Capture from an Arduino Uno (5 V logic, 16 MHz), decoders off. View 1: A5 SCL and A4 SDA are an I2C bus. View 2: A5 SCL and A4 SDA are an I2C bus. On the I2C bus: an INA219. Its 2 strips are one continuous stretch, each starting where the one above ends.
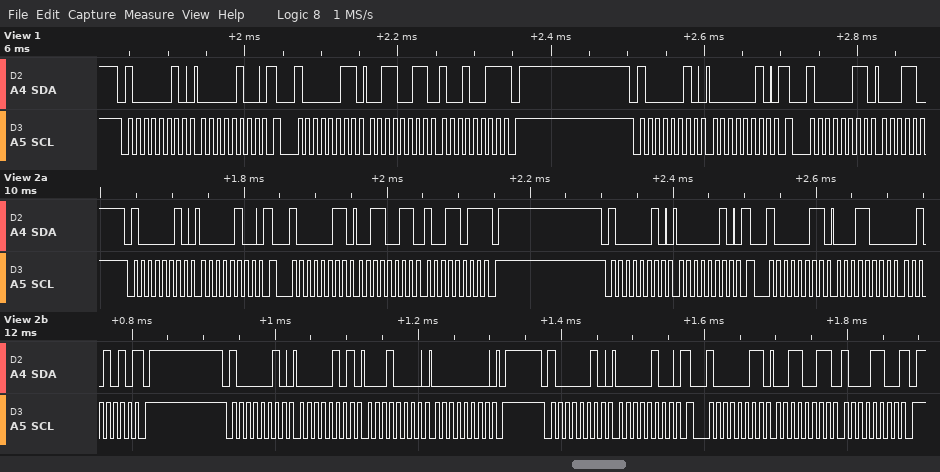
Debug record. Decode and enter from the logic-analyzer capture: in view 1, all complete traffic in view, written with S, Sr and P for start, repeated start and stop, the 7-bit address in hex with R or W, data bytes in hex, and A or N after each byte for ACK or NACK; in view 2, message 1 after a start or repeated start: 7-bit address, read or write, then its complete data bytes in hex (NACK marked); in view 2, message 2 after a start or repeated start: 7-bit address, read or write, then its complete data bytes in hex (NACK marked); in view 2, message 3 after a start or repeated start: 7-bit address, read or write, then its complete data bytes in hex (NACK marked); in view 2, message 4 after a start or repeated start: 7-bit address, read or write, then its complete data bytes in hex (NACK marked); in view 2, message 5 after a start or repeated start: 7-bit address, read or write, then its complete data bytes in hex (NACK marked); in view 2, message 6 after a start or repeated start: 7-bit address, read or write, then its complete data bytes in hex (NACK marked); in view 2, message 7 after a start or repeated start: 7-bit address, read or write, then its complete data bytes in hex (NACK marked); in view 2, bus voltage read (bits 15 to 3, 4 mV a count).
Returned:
S 41W A 04 A Sr 41R A 33 A 93 N P S 41W A 02 A Sr 41R A
0x41 write: 04
0x41 read: 33 9B NACK
0x41 write: 02
0x41 read: 18 2A NACK
0x41 write: 05 10 00
0x41 write: 04
0x41 read: 33 8C NACK
3.092 V
